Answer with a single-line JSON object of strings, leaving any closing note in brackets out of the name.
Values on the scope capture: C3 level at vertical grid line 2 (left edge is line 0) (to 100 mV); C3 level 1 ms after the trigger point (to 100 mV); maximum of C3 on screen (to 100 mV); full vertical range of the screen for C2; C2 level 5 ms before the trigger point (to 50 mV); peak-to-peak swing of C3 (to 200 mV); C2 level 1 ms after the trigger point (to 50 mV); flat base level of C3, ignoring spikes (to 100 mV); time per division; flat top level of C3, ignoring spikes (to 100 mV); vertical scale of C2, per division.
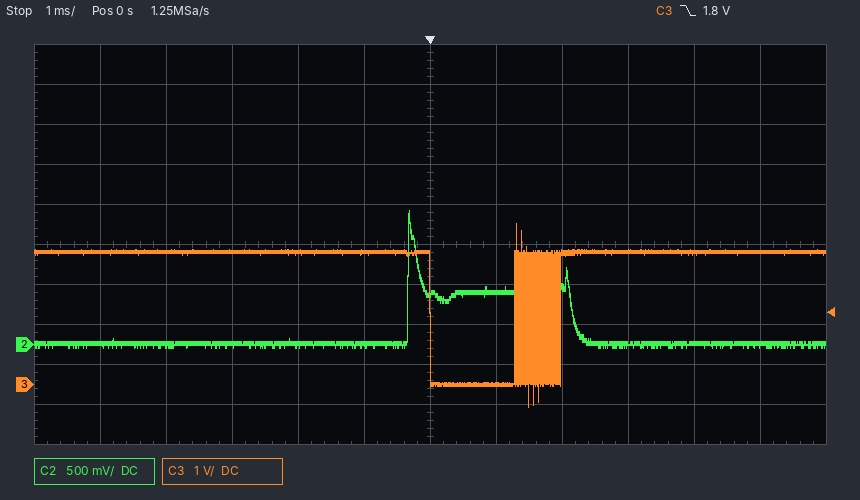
{"C3 level at vertical grid line 2 (left edge is line 0)": "3.3 V", "C3 level 1 ms after the trigger point": "0.0 V", "maximum of C3 on screen": "4.0 V", "full vertical range of the screen for C2": "5 V", "C2 level 5 ms before the trigger point": "0 mV", "peak-to-peak swing of C3": "4.6 V", "C2 level 1 ms after the trigger point": "650 mV", "flat base level of C3, ignoring spikes": "0.0 V", "time per division": "1 ms", "flat top level of C3, ignoring spikes": "3.3 V", "vertical scale of C2, per division": "500 mV"}
